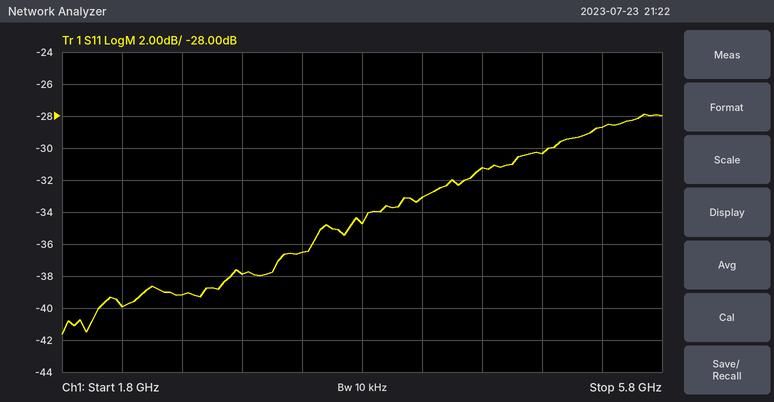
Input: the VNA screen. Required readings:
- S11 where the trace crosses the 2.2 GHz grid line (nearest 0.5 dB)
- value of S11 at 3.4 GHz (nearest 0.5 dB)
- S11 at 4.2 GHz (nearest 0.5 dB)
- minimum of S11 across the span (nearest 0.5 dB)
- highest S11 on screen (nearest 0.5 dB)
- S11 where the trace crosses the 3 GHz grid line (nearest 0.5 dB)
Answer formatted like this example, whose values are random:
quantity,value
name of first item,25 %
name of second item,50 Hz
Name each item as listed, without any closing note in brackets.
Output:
quantity,value
S11 where the trace crosses the 2.2 GHz grid line,-40.0 dB
value of S11 at 3.4 GHz,-36.5 dB
S11 at 4.2 GHz,-33.0 dB
minimum of S11 across the span,-41.5 dB
highest S11 on screen,-28.0 dB
S11 where the trace crosses the 3 GHz grid line,-38.0 dB
